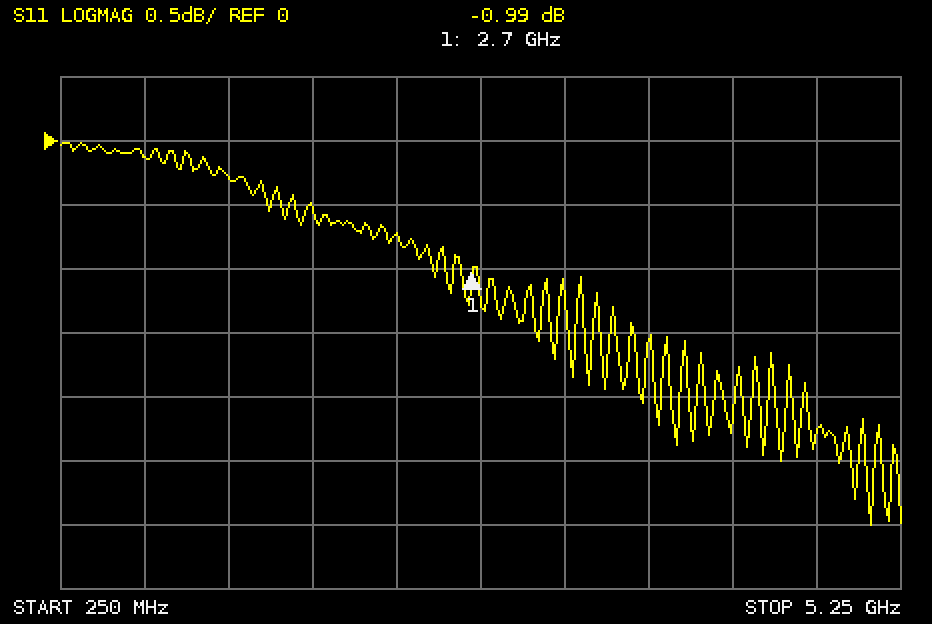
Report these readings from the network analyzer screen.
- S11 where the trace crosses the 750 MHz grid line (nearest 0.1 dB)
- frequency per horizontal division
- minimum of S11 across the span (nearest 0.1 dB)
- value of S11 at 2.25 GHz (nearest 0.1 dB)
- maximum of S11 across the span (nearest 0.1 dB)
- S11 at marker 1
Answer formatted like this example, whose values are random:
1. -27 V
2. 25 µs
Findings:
1. -0.1 dB
2. 500 MHz
3. -3.0 dB
4. -0.7 dB
5. 0.0 dB
6. -0.99 dB
